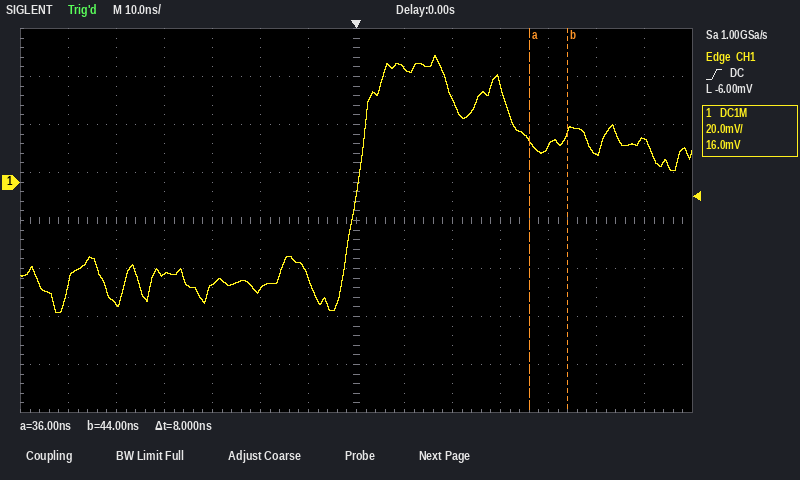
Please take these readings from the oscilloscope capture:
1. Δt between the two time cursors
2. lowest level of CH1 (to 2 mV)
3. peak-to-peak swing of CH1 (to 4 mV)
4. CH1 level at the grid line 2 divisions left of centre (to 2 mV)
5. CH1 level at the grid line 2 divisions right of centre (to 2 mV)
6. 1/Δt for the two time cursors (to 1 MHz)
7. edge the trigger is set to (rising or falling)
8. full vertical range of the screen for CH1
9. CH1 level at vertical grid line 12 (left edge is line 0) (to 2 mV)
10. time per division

8 ns
-54 mV
108 mV
-44 mV
34 mV
125 MHz
rising
160 mV
12 mV
10 ns
